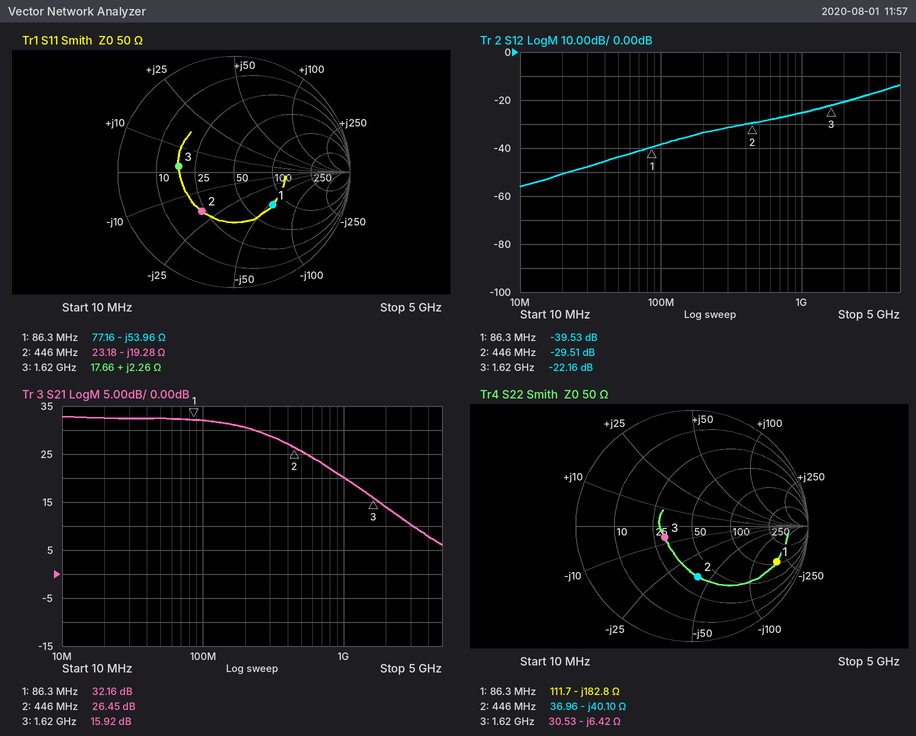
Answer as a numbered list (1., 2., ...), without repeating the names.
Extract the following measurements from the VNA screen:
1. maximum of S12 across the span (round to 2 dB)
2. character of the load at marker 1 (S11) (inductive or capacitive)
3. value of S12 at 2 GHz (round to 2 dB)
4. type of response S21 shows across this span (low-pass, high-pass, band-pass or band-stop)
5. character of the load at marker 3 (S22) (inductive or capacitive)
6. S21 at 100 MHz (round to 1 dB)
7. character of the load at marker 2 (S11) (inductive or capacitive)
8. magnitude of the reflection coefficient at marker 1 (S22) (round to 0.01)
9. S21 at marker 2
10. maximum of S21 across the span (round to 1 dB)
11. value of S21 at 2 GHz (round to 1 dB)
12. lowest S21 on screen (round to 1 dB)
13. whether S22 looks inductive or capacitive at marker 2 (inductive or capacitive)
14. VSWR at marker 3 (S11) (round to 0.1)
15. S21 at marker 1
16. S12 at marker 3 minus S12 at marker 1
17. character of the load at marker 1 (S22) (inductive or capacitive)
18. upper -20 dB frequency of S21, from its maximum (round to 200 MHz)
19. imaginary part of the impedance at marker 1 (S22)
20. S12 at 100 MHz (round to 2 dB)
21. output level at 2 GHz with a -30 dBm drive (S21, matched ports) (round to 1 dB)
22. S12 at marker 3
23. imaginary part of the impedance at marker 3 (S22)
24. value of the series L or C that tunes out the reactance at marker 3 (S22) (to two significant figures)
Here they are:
1. -14 dB
2. capacitive
3. -20 dB
4. low-pass
5. capacitive
6. 32 dB
7. capacitive
8. 0.79
9. 26.45 dB
10. 33 dB
11. 14 dB
12. 6 dB
13. capacitive
14. 2.8
15. 32.16 dB
16. 17.37 dB
17. capacitive
18. 2.2 GHz
19. -182.8 Ω
20. -38 dB
21. -16 dBm
22. -22.16 dB
23. -6.42 Ω
24. 630 pH
